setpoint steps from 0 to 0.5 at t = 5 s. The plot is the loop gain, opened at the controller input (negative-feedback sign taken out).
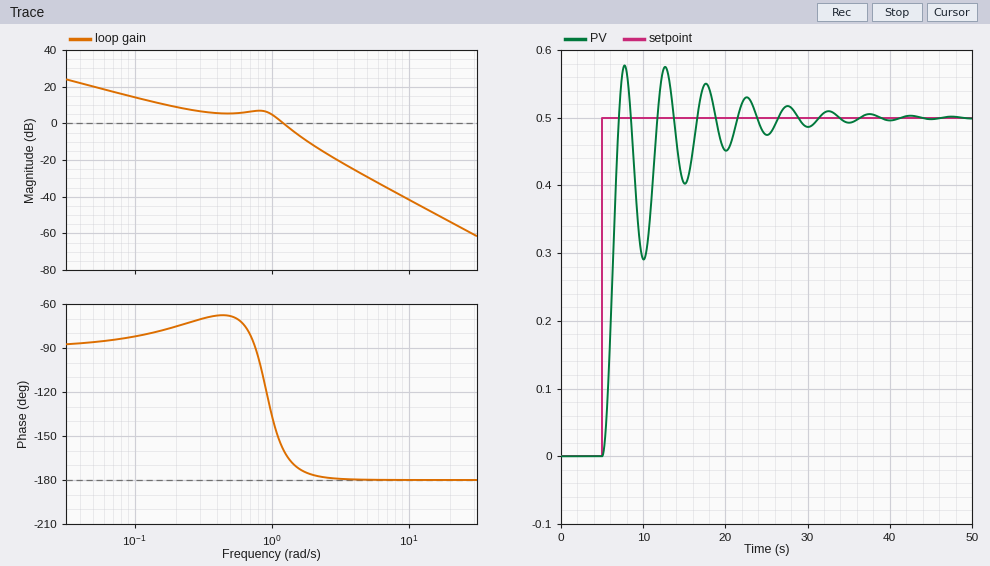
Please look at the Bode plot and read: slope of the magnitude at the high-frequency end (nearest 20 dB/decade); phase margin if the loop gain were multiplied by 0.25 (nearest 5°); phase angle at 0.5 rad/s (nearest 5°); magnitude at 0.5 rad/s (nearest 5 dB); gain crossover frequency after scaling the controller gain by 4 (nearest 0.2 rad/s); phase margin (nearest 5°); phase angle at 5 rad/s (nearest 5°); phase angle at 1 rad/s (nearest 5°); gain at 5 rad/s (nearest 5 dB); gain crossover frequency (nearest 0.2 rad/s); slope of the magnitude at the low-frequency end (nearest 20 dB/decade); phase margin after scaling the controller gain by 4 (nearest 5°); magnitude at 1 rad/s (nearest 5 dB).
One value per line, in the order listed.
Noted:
-40 dB/decade
100°
-70°
5 dB
2.0 rad/s
20°
-180°
-135°
-30 dB
1.2 rad/s
-20 dB/decade
5°
5 dB
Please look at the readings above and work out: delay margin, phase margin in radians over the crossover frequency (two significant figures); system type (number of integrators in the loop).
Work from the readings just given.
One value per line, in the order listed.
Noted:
0.29 s
1
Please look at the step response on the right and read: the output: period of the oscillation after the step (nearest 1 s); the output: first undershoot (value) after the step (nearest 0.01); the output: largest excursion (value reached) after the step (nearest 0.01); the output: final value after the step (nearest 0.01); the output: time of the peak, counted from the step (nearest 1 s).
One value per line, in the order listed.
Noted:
5 s
0.29
0.58
0.50
3 s
